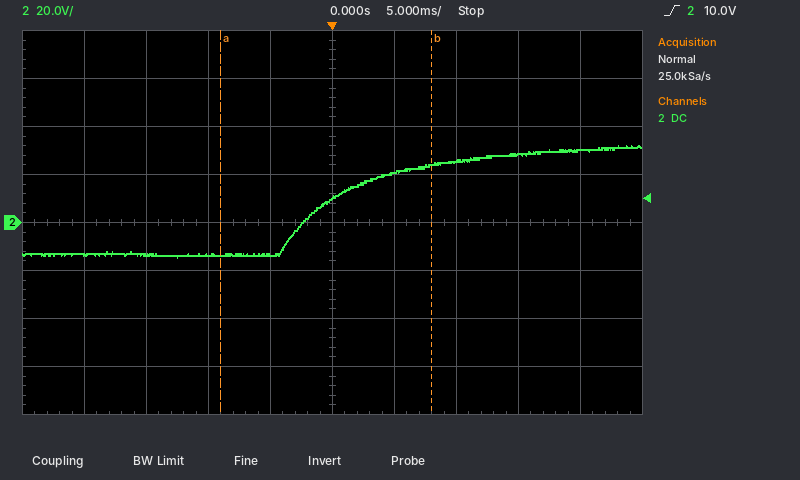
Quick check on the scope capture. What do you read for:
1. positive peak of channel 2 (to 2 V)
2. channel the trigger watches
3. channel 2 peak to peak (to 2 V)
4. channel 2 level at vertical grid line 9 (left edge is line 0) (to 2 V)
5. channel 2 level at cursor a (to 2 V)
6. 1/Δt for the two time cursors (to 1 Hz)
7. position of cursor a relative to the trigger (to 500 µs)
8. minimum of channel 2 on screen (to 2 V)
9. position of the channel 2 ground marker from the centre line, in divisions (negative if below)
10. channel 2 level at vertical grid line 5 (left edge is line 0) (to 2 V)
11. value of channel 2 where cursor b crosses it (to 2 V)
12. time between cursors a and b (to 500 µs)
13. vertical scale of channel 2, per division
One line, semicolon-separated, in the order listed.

32 V; channel 2; 46 V; 30 V; -14 V; 59 Hz; -9.0 ms; -14 V; 0.0 div; 10 V; 24 V; 17.0 ms; 20 V
